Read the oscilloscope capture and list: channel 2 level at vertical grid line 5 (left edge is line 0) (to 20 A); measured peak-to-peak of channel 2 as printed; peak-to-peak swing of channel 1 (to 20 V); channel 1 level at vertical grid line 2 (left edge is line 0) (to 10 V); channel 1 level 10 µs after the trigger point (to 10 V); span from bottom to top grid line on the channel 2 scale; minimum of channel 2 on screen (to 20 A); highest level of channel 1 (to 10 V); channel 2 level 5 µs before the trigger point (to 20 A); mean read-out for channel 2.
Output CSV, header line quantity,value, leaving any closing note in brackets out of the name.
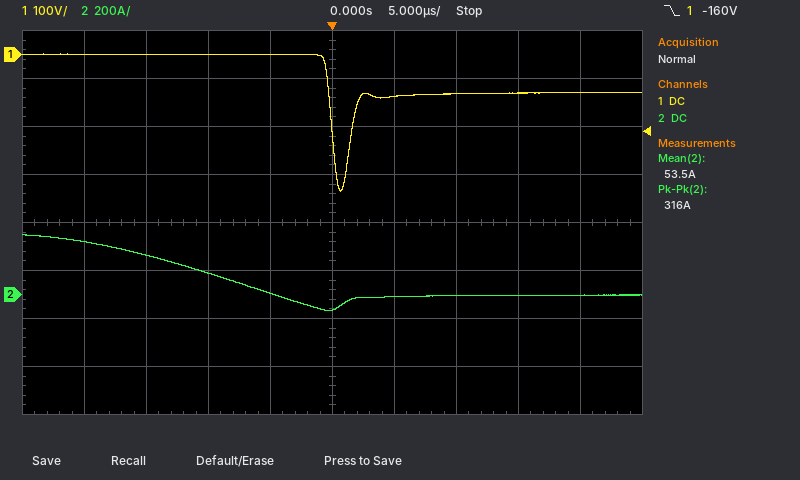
quantity,value
channel 2 level at vertical grid line 5 (left edge is line 0),-60 A
measured peak-to-peak of channel 2 as printed,316 A
peak-to-peak swing of channel 1,280 V
channel 1 level at vertical grid line 2 (left edge is line 0),0 V
channel 1 level 10 µs after the trigger point,-80 V
span from bottom to top grid line on the channel 2 scale,1.6 kA
minimum of channel 2 on screen,-60 A
highest level of channel 1,0 V
channel 2 level 5 µs before the trigger point,0 A
mean read-out for channel 2,53.5 A
